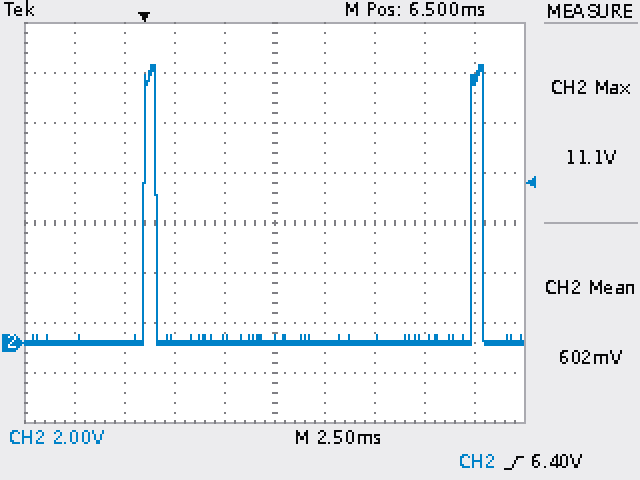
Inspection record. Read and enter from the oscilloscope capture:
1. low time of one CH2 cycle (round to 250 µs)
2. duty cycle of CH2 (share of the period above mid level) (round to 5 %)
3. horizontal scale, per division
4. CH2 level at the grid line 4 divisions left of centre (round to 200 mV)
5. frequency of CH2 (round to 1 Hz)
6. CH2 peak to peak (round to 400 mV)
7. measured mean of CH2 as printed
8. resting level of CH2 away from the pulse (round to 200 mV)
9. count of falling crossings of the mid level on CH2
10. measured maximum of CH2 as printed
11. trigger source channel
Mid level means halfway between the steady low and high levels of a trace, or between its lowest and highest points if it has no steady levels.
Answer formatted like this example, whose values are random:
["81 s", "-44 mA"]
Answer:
["15.75 ms", "5 %", "2.5 ms", "0.0 V", "61 Hz", "11.2 V", "602 mV", "0.0 V", "2", "11.1 V", "CH2"]
